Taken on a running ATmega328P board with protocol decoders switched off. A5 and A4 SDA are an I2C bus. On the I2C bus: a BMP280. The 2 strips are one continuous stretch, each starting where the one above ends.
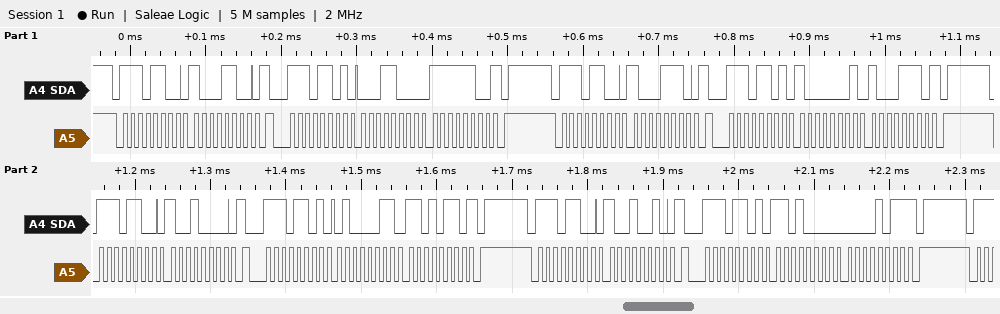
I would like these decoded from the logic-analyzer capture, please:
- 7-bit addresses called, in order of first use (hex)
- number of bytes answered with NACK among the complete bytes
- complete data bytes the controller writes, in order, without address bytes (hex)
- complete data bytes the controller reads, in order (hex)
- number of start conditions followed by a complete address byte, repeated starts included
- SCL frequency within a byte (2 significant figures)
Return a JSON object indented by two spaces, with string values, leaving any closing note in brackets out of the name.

{
  "7-bit addresses called, in order of first use": "0x76",
  "number of bytes answered with NACK among the complete bytes": "4",
  "complete data bytes the controller writes, in order, without address bytes": "8C 8E 90 92",
  "complete data bytes the controller reads, in order": "18 FC 81 8E 43 D6 D0 0B",
  "number of start conditions followed by a complete address byte, repeated starts included": "8",
  "SCL frequency within a byte": "100 kHz"
}
